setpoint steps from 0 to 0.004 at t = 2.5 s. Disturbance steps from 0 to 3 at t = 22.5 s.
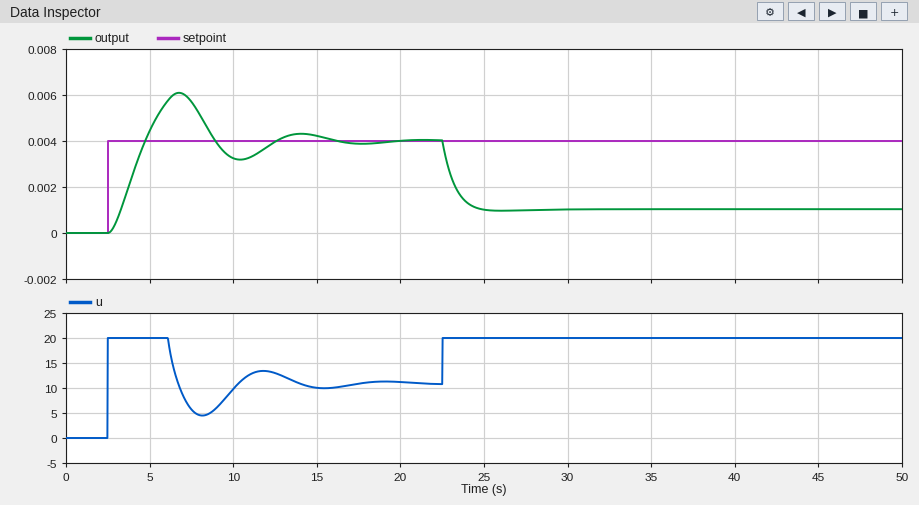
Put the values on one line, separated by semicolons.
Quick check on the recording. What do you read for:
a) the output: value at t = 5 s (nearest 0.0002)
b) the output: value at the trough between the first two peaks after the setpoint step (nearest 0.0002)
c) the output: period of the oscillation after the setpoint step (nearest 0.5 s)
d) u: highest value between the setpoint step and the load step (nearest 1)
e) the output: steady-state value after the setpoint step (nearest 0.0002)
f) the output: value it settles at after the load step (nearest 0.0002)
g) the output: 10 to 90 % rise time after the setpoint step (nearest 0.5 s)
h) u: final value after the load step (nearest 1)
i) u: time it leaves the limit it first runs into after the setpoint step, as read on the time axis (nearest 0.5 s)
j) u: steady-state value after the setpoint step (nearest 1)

0.0044; 0.0032; 7.5 s; 20; 0.0040; 0.0010; 1.5 s; 20; 6.0 s; 11
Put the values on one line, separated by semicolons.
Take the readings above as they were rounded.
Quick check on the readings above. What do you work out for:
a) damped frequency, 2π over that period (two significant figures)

0.84 rad/s
